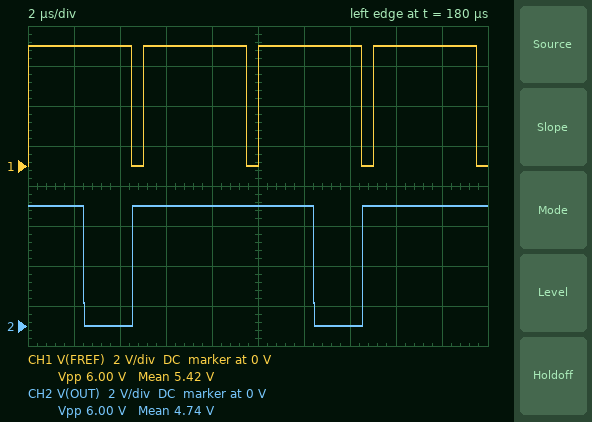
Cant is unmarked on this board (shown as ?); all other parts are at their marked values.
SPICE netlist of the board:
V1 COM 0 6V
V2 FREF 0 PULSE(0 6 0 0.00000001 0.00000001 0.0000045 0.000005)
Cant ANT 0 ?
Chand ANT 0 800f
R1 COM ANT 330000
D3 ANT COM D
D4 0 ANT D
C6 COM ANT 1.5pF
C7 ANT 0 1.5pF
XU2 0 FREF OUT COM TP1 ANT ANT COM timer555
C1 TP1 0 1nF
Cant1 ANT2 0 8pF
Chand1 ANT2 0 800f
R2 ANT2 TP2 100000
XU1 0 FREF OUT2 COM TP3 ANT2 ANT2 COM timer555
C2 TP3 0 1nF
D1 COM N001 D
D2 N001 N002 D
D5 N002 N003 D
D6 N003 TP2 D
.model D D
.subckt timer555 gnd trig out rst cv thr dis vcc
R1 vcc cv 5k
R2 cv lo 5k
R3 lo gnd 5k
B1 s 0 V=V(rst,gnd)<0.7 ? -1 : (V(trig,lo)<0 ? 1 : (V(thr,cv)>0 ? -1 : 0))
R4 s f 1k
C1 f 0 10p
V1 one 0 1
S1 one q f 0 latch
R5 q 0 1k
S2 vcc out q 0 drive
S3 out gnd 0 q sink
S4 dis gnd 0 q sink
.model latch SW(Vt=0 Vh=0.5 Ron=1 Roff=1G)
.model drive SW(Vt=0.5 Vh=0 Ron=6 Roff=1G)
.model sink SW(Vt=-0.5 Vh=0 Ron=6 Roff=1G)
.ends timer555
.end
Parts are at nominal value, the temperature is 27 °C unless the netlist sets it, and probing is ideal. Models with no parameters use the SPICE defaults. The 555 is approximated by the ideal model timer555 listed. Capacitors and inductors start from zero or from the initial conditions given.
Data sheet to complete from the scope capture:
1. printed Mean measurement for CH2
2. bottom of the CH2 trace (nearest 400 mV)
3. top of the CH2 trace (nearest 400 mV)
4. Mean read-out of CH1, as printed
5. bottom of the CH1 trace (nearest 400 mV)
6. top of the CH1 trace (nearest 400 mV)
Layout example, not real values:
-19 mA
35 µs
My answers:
4.74 V
0 V
6.0 V
5.42 V
0 V
6.0 V
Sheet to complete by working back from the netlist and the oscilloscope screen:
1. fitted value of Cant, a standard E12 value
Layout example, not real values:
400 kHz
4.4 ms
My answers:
18 pF
